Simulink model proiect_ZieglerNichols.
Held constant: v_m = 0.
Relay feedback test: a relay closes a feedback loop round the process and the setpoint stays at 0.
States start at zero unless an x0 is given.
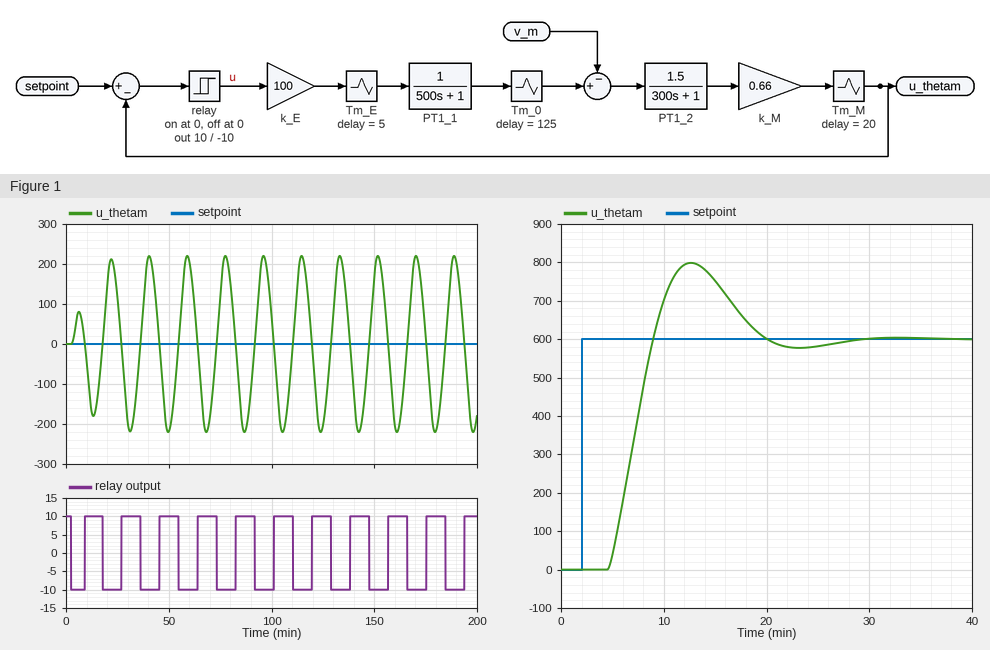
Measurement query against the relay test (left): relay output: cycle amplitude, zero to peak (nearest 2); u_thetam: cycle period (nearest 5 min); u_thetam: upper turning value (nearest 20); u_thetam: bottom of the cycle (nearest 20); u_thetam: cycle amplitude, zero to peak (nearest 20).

10
20 min
220
-220
220
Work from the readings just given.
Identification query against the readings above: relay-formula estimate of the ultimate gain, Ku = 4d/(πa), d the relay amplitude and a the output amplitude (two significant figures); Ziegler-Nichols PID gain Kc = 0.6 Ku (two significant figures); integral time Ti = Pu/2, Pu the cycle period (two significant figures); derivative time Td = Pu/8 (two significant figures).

0.058
0.035
10 min
2.5 min
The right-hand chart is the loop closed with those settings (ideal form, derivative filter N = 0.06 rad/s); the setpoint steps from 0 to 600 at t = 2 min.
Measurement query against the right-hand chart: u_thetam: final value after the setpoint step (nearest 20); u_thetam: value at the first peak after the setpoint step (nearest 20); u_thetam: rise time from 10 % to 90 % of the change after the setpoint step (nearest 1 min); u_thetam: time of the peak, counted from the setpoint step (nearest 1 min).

600
800
3 min
11 min
